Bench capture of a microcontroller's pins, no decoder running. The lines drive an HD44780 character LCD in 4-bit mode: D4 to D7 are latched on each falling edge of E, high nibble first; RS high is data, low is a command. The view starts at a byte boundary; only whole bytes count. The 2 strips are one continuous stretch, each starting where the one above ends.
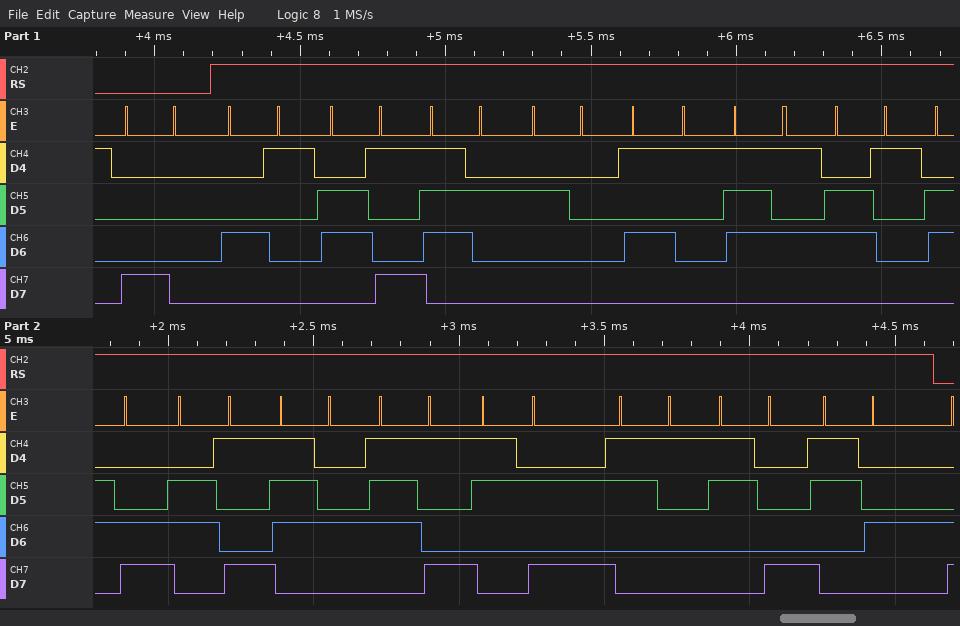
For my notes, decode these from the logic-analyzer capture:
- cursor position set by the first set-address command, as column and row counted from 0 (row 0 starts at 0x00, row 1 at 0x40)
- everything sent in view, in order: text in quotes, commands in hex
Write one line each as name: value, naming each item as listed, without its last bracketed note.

cursor position set by the first set-address command, as column and row counted from 0: column 0, row 0
everything sent in view, in order: text in quotes, commands in hex: 0x80 "Air Quality:184"
